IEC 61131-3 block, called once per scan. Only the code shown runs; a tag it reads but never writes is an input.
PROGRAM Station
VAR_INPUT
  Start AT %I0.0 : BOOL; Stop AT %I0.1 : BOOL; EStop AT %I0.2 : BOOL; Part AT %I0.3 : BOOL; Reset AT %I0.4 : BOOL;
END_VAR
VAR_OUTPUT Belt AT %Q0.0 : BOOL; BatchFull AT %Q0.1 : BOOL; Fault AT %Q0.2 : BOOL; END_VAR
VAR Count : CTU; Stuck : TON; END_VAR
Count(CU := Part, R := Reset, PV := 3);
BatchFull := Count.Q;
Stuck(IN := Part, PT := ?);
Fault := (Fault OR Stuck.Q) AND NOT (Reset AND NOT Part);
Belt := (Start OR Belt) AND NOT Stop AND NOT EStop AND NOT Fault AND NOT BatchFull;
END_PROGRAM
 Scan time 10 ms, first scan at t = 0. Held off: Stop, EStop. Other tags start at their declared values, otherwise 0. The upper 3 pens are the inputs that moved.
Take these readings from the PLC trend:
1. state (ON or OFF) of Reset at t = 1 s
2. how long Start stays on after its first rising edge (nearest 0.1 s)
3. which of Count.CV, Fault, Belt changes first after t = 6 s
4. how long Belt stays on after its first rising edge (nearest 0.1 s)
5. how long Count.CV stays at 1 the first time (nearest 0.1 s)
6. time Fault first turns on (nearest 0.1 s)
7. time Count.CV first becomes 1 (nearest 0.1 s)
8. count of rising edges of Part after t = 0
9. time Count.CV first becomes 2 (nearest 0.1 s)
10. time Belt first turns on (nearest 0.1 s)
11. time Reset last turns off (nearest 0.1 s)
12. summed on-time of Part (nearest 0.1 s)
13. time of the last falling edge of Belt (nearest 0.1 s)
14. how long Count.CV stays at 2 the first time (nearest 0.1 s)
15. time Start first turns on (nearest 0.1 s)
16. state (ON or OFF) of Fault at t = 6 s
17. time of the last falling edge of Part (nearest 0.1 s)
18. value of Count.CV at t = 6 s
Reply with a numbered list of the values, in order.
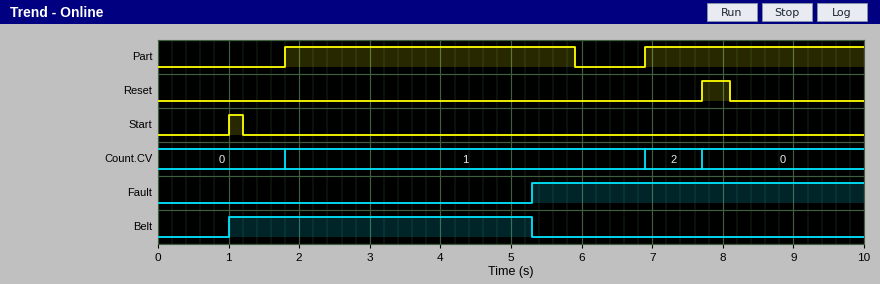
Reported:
1. OFF
2. 0.2 s
3. Count.CV
4. 4.3 s
5. 5.1 s
6. 5.3 s
7. 1.8 s
8. 2
9. 6.9 s
10. 1.0 s
11. 8.1 s
12. 7.2 s
13. 5.3 s
14. 0.8 s
15. 1.0 s
16. ON
17. 5.9 s
18. 1
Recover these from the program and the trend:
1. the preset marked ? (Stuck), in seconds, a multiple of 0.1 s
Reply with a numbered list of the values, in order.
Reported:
1. 3.5 s
